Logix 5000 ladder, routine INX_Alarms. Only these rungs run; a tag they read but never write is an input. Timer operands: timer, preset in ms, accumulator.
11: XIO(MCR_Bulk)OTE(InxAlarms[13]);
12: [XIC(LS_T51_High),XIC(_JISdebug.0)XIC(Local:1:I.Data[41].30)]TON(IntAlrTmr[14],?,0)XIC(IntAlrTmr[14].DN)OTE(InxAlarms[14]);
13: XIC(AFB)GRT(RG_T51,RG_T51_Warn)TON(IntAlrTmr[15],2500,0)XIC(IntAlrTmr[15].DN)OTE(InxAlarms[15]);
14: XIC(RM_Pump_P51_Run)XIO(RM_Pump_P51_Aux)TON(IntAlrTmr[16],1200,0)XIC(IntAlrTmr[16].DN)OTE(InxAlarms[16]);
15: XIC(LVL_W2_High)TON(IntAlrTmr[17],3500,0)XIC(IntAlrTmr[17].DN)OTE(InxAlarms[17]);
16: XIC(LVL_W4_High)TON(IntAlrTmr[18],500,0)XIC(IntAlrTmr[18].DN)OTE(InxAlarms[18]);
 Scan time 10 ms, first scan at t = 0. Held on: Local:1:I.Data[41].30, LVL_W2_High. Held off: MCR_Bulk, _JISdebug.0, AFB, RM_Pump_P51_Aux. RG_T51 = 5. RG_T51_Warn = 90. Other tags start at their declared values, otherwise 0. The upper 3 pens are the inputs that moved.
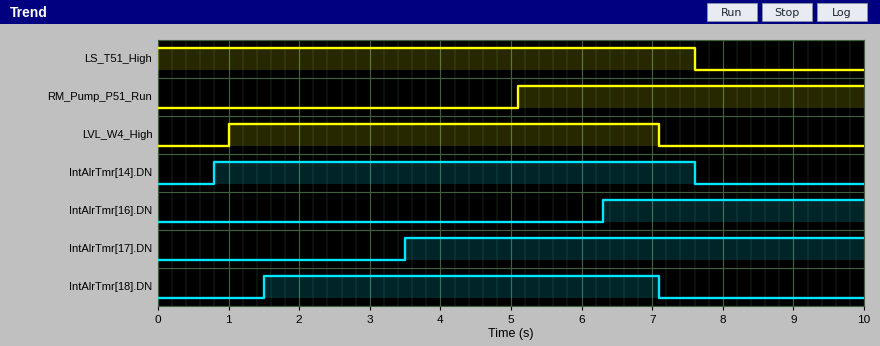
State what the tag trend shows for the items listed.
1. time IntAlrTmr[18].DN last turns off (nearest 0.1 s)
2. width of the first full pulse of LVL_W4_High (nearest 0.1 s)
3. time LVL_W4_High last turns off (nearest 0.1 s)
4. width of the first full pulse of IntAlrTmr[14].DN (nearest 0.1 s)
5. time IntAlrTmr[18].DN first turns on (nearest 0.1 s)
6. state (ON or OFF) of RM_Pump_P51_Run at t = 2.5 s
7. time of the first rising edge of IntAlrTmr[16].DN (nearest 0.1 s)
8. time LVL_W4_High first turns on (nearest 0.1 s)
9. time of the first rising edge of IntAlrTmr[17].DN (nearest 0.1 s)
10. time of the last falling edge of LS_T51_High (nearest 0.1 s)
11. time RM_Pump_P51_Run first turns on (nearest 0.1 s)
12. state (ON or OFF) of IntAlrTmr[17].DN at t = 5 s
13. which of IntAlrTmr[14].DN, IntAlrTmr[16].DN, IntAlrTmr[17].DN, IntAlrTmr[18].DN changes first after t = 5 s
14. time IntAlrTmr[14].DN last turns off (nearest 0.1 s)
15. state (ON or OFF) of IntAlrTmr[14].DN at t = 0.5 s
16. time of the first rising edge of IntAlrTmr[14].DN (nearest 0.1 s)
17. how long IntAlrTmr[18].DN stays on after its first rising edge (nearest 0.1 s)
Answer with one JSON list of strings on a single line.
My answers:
["7.1 s", "6.1 s", "7.1 s", "6.8 s", "1.5 s", "OFF", "6.3 s", "1.0 s", "3.5 s", "7.6 s", "5.1 s", "ON", "IntAlrTmr[16].DN", "7.6 s", "OFF", "0.8 s", "5.6 s"]
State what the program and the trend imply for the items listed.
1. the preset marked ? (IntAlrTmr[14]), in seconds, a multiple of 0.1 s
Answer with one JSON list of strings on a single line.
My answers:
["0.8 s"]
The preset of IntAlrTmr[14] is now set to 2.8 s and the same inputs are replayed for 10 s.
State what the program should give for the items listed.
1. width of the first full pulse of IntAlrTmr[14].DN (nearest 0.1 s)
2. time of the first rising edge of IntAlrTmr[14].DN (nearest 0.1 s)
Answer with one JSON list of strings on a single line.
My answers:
["4.8 s", "2.8 s"]
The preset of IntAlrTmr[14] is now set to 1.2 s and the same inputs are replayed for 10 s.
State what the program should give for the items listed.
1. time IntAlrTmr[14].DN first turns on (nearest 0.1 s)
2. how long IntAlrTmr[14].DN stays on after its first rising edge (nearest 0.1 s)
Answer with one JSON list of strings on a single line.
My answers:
["1.2 s", "6.4 s"]
